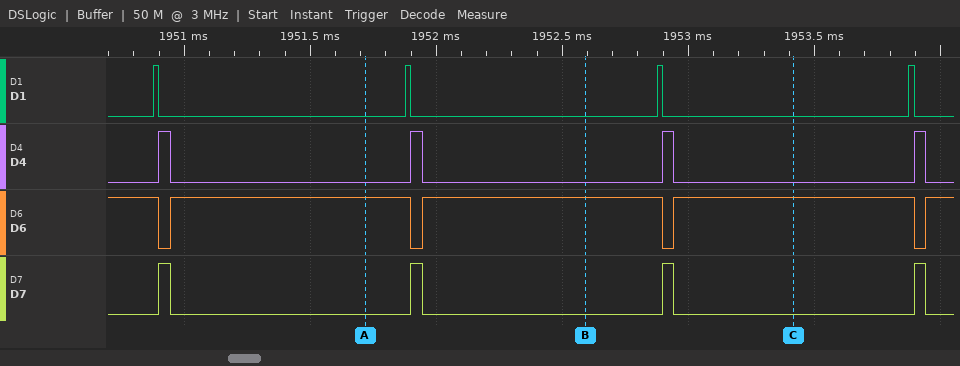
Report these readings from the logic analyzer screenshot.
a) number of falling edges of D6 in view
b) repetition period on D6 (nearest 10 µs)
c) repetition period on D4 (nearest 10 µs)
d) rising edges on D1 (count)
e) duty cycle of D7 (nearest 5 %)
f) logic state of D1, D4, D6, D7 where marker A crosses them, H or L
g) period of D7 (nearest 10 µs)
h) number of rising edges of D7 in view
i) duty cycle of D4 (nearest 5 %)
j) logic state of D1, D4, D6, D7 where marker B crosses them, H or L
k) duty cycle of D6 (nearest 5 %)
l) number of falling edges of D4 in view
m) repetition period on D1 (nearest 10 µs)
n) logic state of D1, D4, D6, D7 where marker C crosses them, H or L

4
1000 µs
1000 µs
4
5 %
D1=L, D4=L, D6=H, D7=L
1000 µs
4
5 %
D1=L, D4=L, D6=H, D7=L
95 %
4
1000 µs
D1=L, D4=L, D6=H, D7=L
